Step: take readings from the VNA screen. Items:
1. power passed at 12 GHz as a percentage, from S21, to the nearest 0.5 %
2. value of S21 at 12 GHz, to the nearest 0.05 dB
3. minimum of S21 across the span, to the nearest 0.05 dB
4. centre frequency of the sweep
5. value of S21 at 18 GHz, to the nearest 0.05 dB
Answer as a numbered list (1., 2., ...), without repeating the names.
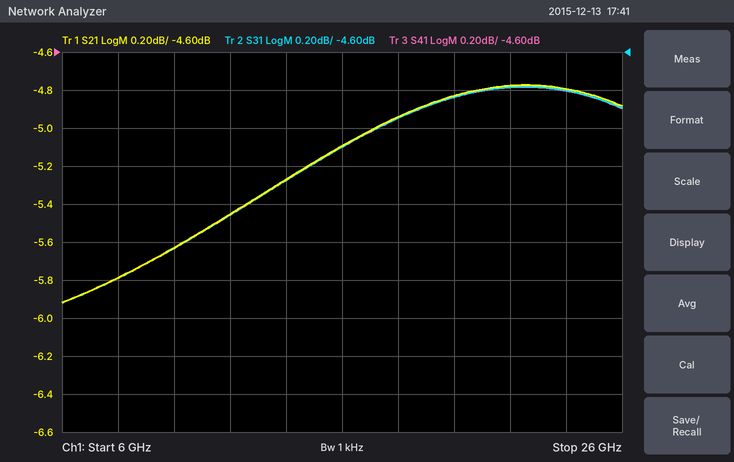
1. 28.5 %
2. -5.45 dB
3. -5.90 dB
4. 16 GHz
5. -4.95 dB
